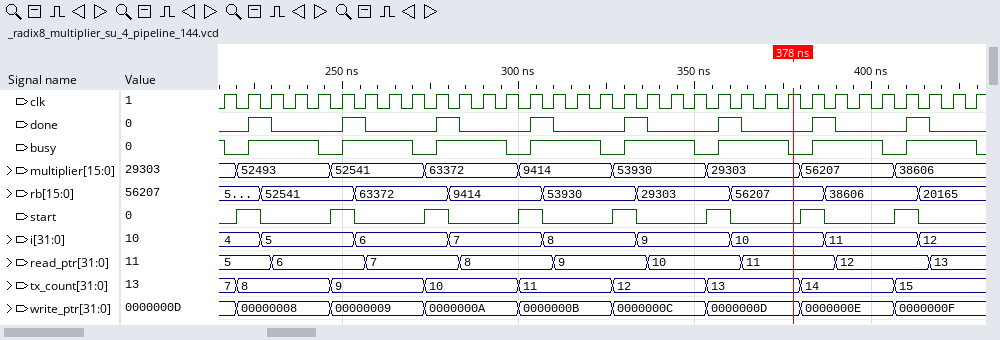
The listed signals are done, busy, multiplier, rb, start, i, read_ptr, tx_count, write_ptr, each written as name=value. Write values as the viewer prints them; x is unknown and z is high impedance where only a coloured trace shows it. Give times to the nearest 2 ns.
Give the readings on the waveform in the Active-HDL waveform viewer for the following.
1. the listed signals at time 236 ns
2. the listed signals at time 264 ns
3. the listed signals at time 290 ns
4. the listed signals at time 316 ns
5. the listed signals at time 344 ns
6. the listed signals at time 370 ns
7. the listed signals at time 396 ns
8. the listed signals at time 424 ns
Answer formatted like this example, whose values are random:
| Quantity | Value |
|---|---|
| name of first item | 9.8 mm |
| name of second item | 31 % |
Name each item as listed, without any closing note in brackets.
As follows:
| Quantity | Value |
|---|---|
| the listed signals at time 236 ns | done=0, busy=1, multiplier=52493, rb=52541, start=0, i=5, read_ptr=6, tx_count=8, write_ptr=00000008 |
| the listed signals at time 264 ns | done=0, busy=1, multiplier=52541, rb=63372, start=0, i=6, read_ptr=7, tx_count=9, write_ptr=00000009 |
| the listed signals at time 290 ns | done=0, busy=1, multiplier=63372, rb=9414, start=0, i=7, read_ptr=8, tx_count=10, write_ptr=0000000A |
| the listed signals at time 316 ns | done=0, busy=1, multiplier=9414, rb=53930, start=0, i=8, read_ptr=9, tx_count=11, write_ptr=0000000B |
| the listed signals at time 344 ns | done=0, busy=1, multiplier=53930, rb=29303, start=0, i=9, read_ptr=10, tx_count=12, write_ptr=0000000C |
| the listed signals at time 370 ns | done=0, busy=1, multiplier=29303, rb=56207, start=0, i=10, read_ptr=11, tx_count=13, write_ptr=0000000D |
| the listed signals at time 396 ns | done=0, busy=1, multiplier=56207, rb=38606, start=0, i=11, read_ptr=12, tx_count=14, write_ptr=0000000E |
| the listed signals at time 424 ns | done=0, busy=1, multiplier=38606, rb=20165, start=0, i=12, read_ptr=13, tx_count=15, write_ptr=0000000F |
